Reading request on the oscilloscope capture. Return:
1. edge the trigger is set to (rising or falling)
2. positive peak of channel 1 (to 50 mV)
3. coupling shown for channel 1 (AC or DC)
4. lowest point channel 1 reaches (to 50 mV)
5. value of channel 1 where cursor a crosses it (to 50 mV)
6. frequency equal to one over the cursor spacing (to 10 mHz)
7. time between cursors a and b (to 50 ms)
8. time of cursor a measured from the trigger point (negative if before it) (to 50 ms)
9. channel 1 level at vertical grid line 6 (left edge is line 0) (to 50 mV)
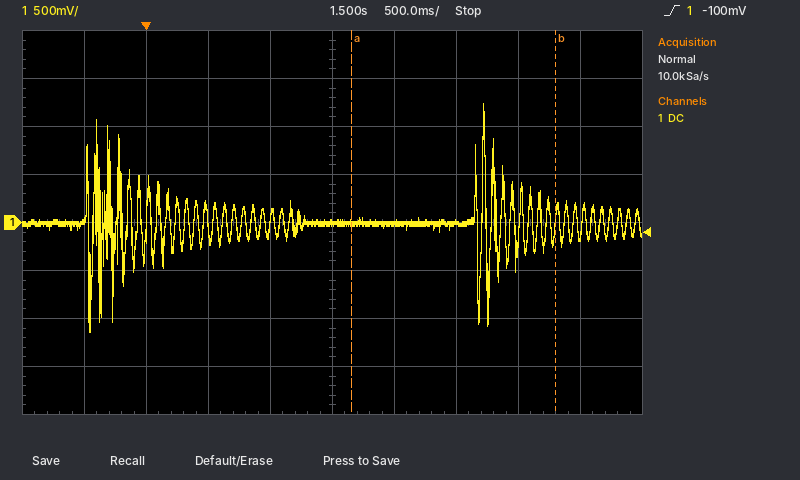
rising
1.25 V
DC
-1.15 V
0 mV
610 mHz
1.65 s
+1.65 s
0 mV
